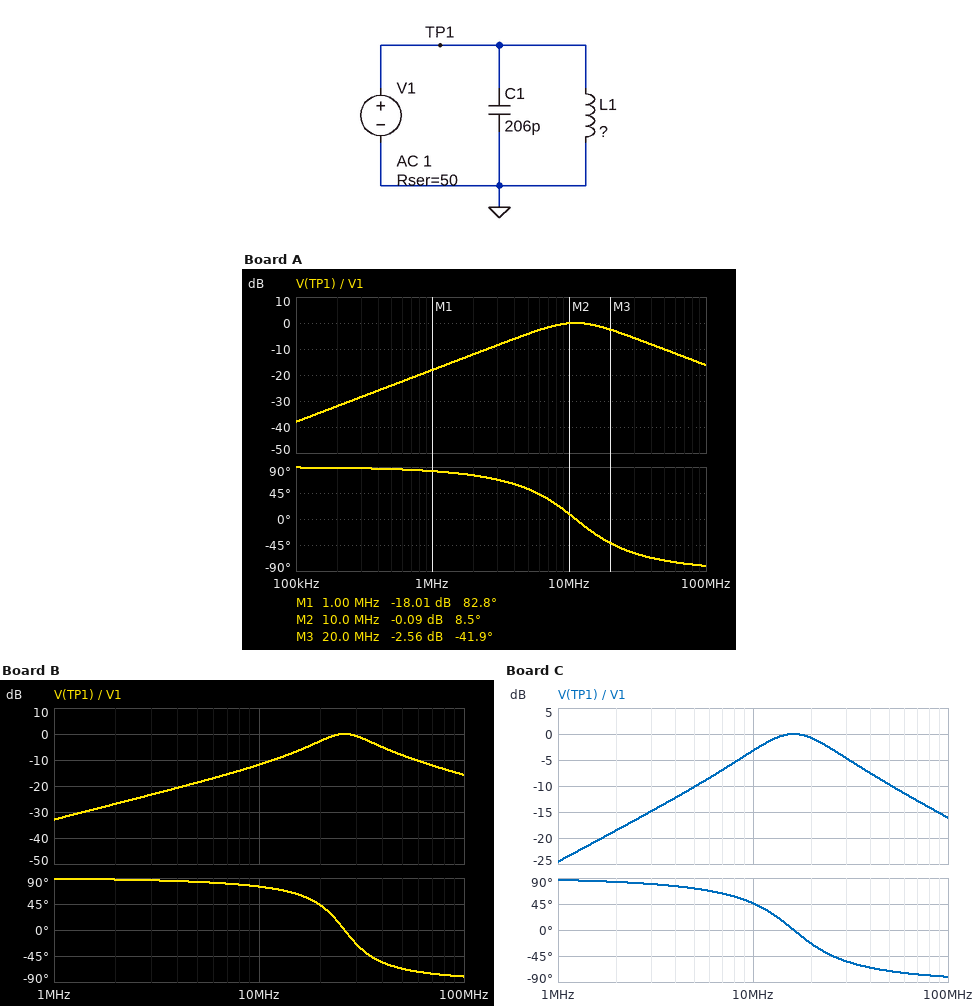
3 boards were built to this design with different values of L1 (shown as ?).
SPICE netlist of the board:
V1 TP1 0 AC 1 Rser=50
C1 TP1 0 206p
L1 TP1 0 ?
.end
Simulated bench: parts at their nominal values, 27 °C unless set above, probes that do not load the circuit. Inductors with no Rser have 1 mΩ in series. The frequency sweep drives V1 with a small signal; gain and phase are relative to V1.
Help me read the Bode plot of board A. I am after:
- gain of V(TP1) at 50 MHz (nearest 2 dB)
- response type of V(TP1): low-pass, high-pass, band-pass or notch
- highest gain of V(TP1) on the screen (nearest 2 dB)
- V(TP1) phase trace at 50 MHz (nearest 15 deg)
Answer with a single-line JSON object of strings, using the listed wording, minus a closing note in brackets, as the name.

{"gain of V(TP1) at 50 MHz": "-10 dB", "response type of V(TP1): low-pass, high-pass, band-pass or notch": "band-pass", "highest gain of V(TP1) on the screen": "0 dB", "V(TP1) phase trace at 50 MHz": "-75 deg"}
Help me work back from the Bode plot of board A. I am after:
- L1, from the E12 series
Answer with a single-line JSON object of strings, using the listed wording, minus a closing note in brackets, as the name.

{"L1, from the E12 series": "1 µH"}
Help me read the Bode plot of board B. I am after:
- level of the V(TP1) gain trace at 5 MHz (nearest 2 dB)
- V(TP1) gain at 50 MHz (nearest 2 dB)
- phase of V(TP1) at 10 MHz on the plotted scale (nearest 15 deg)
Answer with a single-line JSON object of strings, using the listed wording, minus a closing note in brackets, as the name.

{"level of the V(TP1) gain trace at 5 MHz": "-18 dB", "V(TP1) gain at 50 MHz": "-8 dB", "phase of V(TP1) at 10 MHz on the plotted scale": "75 deg"}
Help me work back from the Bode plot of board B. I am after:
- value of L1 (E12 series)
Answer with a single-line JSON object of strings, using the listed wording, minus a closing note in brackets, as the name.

{"value of L1": "180 nH"}
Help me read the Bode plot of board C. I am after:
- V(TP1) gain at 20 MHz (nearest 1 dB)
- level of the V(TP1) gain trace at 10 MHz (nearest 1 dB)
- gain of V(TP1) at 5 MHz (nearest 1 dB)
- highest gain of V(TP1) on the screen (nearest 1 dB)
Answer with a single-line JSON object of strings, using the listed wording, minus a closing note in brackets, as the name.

{"V(TP1) gain at 20 MHz": "-1 dB", "level of the V(TP1) gain trace at 10 MHz": "-3 dB", "gain of V(TP1) at 5 MHz": "-10 dB", "highest gain of V(TP1) on the screen": "0 dB"}
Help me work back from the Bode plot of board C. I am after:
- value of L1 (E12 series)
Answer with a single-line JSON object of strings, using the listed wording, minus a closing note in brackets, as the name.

{"value of L1": "470 nH"}
